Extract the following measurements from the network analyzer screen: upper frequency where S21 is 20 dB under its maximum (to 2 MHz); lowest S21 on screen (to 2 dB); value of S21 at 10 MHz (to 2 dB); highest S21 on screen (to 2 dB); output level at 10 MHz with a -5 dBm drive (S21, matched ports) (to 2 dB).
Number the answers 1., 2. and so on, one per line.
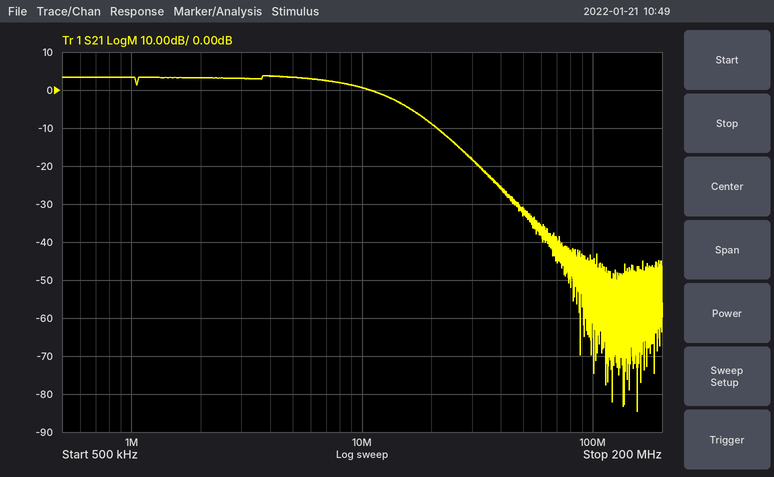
1. 28 MHz
2. -84 dB
3. 0 dB
4. 4 dB
5. -4 dBm
